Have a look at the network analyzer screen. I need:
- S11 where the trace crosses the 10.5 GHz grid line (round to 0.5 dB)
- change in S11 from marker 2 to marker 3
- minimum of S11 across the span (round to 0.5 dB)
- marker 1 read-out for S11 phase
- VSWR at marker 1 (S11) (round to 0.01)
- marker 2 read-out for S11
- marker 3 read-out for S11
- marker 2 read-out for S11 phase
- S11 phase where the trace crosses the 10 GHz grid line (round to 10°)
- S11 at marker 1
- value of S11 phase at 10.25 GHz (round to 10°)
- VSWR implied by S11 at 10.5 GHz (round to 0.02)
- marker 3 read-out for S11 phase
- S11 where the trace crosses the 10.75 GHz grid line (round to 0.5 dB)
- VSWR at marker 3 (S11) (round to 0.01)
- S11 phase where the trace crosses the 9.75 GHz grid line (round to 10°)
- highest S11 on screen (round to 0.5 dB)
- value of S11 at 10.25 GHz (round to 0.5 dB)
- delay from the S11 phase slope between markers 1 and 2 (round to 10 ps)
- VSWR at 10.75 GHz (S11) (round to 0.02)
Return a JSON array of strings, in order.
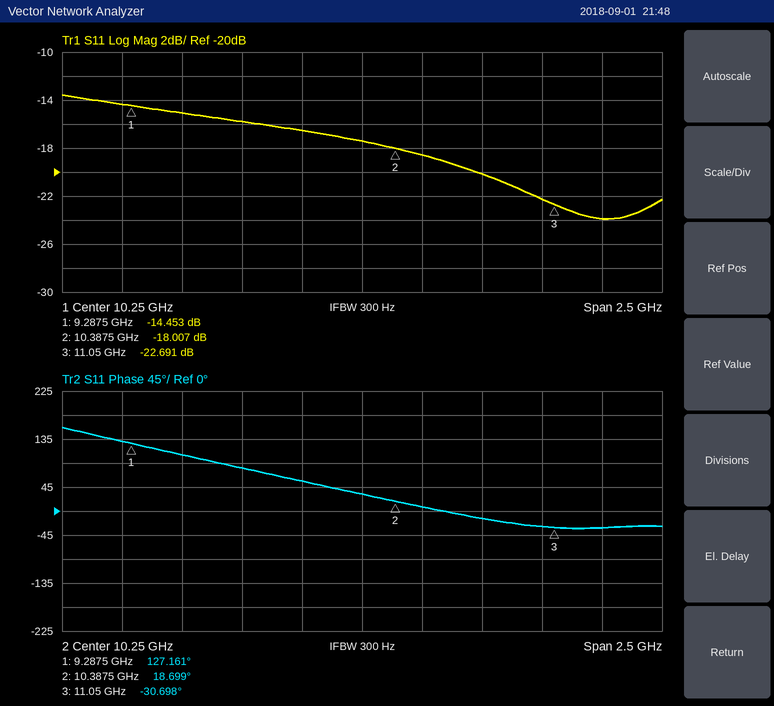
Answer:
["-18.5 dB", "-4.684 dB", "-24.0 dB", "127.161°", "1.47", "-18.007 dB", "-22.691 dB", "18.699°", "60°", "-14.453 dB", "30°", "1.26", "-30.698°", "-20.0 dB", "1.16", "80°", "-13.5 dB", "-17.5 dB", "270 ps", "1.22"]
